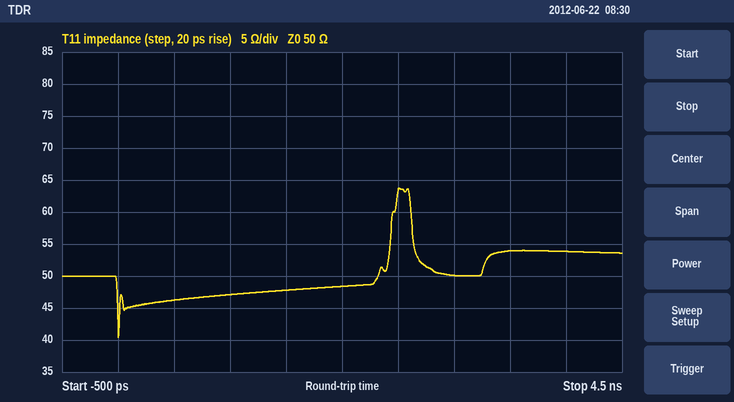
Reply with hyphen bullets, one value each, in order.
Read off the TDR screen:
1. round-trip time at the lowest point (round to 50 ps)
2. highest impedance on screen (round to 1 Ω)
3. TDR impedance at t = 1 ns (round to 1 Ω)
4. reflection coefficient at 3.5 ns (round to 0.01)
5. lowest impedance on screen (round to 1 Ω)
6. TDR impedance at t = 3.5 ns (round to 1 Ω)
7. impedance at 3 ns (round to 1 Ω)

- 0 ps
- 64 Ω
- 47 Ω
- +0.04
- 40 Ω
- 54 Ω
- 50 Ω
